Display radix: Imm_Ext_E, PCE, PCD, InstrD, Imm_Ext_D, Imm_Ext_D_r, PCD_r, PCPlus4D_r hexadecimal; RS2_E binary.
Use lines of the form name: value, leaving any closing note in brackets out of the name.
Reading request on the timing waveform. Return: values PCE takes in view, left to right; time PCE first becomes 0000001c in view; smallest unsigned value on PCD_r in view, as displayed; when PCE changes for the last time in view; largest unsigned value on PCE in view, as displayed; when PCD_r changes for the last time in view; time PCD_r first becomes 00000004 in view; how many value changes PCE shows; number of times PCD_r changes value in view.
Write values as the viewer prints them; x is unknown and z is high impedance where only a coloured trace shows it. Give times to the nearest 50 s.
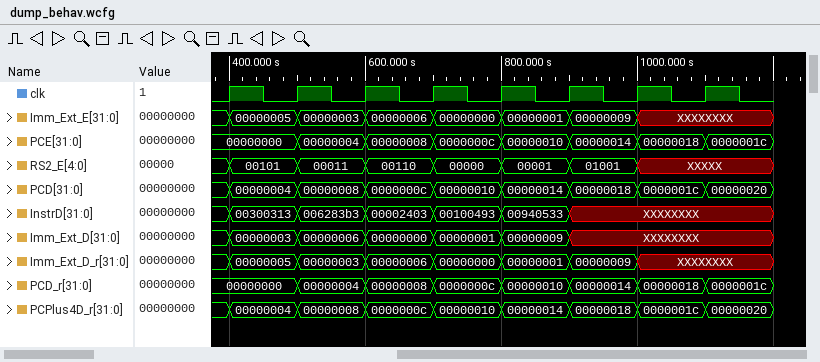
values PCE takes in view, left to right: 00000000, 00000004, 00000008, 0000000c, 00000010, 00000014, 00000018, 0000001c
time PCE first becomes 0000001c in view: 1100 s
smallest unsigned value on PCD_r in view, as displayed: 00000000
when PCE changes for the last time in view: 1100 s
largest unsigned value on PCE in view, as displayed: 0000001c
when PCD_r changes for the last time in view: 1100 s
time PCD_r first becomes 00000004 in view: 500 s
how many value changes PCE shows: 7
number of times PCD_r changes value in view: 7
